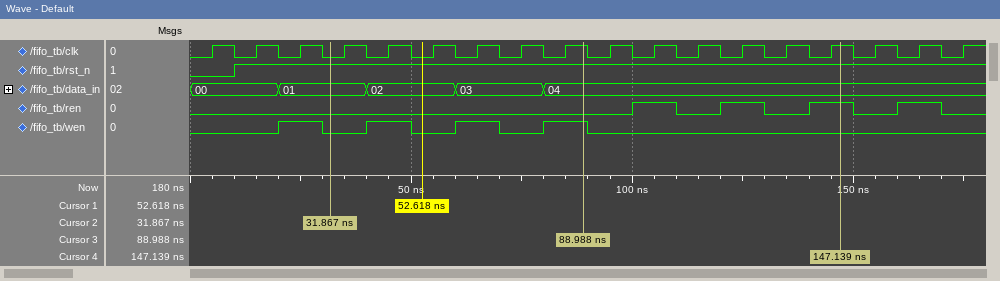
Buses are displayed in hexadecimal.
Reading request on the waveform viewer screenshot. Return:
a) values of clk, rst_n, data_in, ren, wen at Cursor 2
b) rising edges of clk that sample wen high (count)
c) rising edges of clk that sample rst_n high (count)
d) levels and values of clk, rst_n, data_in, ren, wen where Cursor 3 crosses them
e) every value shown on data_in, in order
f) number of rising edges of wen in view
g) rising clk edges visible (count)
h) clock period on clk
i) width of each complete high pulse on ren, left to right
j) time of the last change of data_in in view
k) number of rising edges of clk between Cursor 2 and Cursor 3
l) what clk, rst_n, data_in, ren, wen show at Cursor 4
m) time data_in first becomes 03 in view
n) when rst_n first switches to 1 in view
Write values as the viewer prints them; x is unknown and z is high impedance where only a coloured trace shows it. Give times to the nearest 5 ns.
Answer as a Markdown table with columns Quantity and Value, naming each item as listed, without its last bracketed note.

| Quantity | Value |
|---|---|
| values of clk, rst_n, data_in, ren, wen at Cursor 2 | clk=0, rst_n=1, data_in=01, ren=0, wen=0 |
| rising edges of clk that sample wen high | 4 |
| rising edges of clk that sample rst_n high | 17 |
| levels and values of clk, rst_n, data_in, ren, wen where Cursor 3 crosses them | clk=1, rst_n=1, data_in=04, ren=0, wen=1 |
| every value shown on data_in, in order | 00, 01, 02, 03, 04 |
| number of rising edges of wen in view | 4 |
| rising clk edges visible | 18 |
| clock period on clk | 10 ns |
| width of each complete high pulse on ren, left to right | 10 ns, 10 ns, 10 ns, 10 ns |
| time of the last change of data_in in view | 80 ns |
| number of rising edges of clk between Cursor 2 and Cursor 3 | 6 |
| what clk, rst_n, data_in, ren, wen show at Cursor 4 | clk=1, rst_n=1, data_in=04, ren=1, wen=0 |
| time data_in first becomes 03 in view | 60 ns |
| when rst_n first switches to 1 in view | 10 ns |
